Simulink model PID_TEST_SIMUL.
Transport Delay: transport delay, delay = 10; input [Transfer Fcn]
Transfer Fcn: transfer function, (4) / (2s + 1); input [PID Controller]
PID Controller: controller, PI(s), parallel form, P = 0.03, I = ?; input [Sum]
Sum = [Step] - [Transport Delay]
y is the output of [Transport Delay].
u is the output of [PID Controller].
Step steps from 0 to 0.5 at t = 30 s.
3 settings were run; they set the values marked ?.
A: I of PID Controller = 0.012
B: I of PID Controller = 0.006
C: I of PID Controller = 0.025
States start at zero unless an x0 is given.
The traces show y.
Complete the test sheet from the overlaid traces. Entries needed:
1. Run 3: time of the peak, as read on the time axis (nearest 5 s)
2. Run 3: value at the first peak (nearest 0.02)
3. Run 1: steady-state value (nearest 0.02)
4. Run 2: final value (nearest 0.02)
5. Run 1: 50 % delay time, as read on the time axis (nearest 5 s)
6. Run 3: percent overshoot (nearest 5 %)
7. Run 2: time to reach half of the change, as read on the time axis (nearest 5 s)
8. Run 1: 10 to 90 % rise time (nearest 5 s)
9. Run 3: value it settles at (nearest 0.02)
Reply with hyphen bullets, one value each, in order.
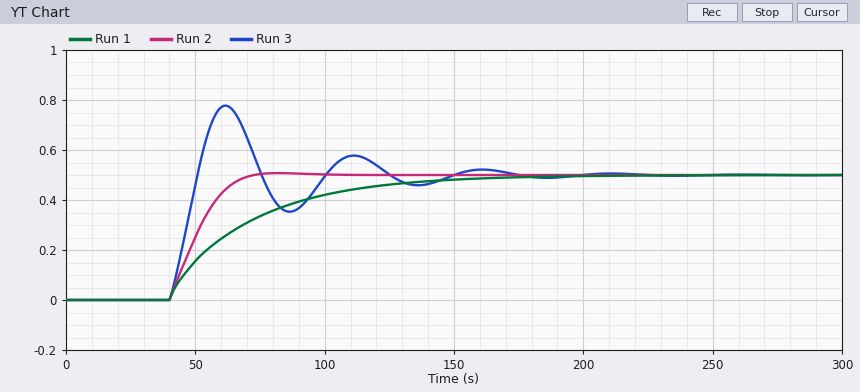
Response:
- 60 s
- 0.78
- 0.50
- 0.50
- 60 s
- 55 %
- 50 s
- 75 s
- 0.50
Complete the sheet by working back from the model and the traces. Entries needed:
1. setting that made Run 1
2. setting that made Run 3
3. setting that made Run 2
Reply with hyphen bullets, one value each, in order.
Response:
- B
- C
- A
